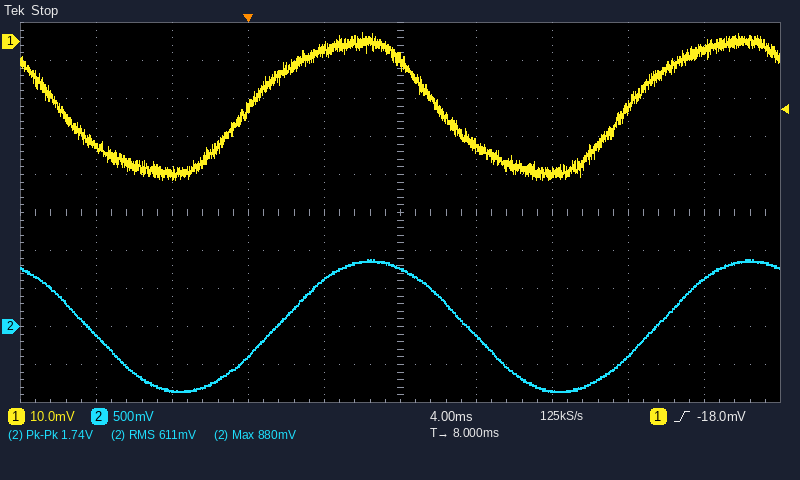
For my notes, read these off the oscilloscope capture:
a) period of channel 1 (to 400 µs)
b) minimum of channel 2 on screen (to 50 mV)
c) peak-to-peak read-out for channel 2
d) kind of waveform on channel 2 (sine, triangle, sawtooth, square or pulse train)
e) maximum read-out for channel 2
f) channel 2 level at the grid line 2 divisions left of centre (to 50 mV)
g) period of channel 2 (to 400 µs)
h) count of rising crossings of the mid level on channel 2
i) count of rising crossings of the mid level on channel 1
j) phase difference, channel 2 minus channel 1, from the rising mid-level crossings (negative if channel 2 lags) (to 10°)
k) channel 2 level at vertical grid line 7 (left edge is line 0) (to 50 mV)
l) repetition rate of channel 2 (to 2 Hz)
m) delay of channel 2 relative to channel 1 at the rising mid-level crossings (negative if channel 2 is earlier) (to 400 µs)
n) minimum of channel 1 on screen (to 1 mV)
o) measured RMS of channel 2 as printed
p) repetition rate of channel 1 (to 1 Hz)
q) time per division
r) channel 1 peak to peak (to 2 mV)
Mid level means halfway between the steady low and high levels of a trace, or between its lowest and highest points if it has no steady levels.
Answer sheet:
20.0 ms
-850 mV
1.74 V
sine
880 mV
-400 mV
20.0 ms
2
2
-30°
-850 mV
50 Hz
+1.6 ms
-36 mV
611 mV
50 Hz
4 ms
38 mV
